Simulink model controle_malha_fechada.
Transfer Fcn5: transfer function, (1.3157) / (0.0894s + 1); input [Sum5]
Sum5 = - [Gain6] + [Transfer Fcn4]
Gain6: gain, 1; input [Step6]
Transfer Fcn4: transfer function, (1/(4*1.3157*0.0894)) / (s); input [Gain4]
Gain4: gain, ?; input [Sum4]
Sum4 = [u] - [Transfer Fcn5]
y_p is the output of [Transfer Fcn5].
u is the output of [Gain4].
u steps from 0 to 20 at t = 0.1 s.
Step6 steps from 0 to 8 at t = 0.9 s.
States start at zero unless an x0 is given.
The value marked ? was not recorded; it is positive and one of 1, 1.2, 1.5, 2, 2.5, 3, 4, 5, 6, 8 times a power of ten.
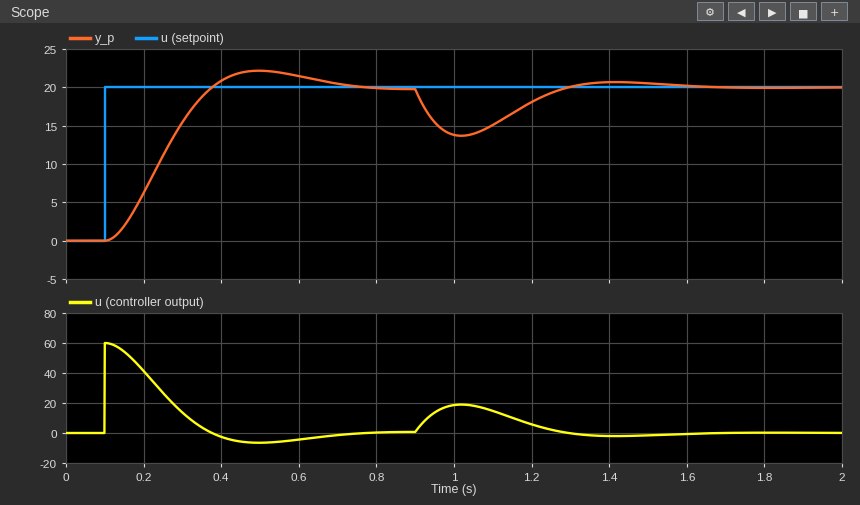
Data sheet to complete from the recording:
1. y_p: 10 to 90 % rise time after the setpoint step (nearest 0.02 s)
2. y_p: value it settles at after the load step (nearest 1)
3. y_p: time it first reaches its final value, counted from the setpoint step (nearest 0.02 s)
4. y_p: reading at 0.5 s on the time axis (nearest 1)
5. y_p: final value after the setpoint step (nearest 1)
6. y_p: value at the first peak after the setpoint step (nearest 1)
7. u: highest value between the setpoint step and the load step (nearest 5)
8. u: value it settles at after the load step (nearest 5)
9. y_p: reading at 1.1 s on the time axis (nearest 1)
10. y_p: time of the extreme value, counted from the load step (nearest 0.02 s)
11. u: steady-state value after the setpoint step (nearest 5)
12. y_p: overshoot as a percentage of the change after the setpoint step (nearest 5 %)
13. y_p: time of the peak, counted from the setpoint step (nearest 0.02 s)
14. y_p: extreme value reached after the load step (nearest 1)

0.18 s
20
0.28 s
22
20
22
60
0
15
0.12 s
0
10 %
0.40 s
14
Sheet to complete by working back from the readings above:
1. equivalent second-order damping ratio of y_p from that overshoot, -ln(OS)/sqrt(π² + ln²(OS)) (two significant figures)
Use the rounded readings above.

0.59
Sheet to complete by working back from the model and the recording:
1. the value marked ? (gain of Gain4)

3
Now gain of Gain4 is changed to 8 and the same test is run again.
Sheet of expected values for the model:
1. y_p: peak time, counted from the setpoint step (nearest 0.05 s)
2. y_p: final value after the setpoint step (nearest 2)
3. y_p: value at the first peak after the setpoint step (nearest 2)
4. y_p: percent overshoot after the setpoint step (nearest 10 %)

0.20 s
20
26
30 %
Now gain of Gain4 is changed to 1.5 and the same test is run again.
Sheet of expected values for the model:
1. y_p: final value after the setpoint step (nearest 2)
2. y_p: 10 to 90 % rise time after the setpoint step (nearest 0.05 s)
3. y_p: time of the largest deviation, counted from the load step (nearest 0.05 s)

20
0.35 s
0.15 s
